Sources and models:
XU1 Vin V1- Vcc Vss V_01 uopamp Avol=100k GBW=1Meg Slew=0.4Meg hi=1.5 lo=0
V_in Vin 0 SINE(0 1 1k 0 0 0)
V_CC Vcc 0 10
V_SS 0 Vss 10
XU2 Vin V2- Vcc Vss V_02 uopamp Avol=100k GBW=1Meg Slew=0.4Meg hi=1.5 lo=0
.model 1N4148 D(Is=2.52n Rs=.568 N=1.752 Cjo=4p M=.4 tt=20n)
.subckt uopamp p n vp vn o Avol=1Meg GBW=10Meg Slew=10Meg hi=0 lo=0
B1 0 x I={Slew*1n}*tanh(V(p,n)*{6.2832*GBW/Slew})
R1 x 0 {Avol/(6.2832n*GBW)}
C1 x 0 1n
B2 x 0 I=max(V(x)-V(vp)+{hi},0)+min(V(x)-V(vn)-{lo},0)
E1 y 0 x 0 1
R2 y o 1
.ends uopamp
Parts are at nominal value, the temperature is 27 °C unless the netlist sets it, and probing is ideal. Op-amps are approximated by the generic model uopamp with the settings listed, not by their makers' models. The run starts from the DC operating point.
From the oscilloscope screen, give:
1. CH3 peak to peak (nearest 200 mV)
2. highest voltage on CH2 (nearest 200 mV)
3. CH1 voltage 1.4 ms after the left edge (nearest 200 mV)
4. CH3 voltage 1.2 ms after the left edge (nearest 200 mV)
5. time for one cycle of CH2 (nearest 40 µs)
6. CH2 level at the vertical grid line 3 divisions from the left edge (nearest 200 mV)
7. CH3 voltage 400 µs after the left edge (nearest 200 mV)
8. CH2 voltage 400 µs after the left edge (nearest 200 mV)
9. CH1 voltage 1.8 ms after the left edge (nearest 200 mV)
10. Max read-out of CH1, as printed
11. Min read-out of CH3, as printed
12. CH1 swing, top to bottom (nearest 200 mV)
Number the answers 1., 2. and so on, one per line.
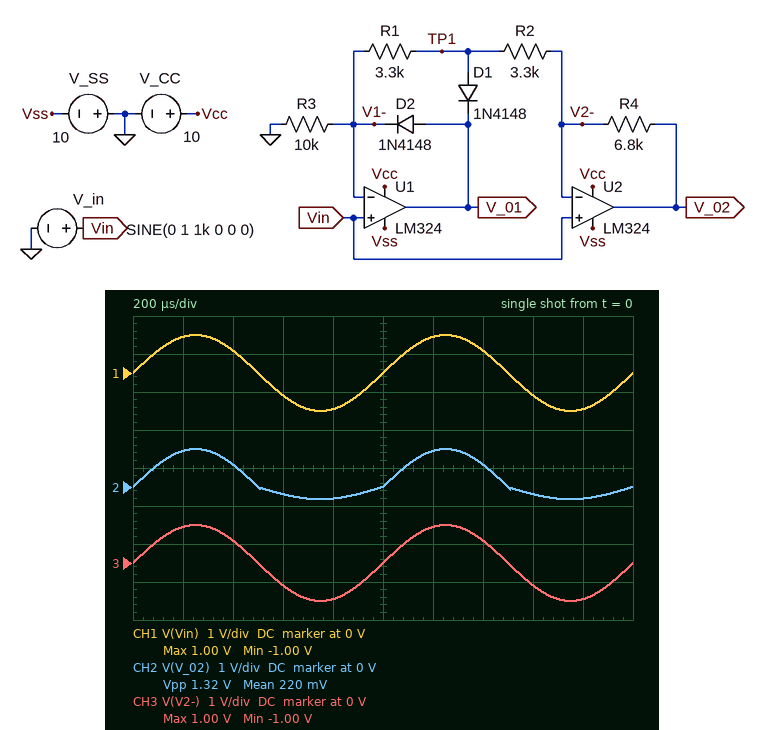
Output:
1. 2.0 V
2. 1.0 V
3. 600 mV
4. 1.0 V
5. 1.00 ms
6. -200 mV
7. 600 mV
8. 600 mV
9. -1.0 V
10. 1.00 V
11. -1.00 V
12. 2.0 V
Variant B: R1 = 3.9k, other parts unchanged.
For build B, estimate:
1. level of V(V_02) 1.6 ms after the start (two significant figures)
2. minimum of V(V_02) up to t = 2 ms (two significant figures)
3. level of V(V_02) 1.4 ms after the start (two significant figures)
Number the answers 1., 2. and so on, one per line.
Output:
1. -120 mV
2. -200 mV
3. 590 mV
